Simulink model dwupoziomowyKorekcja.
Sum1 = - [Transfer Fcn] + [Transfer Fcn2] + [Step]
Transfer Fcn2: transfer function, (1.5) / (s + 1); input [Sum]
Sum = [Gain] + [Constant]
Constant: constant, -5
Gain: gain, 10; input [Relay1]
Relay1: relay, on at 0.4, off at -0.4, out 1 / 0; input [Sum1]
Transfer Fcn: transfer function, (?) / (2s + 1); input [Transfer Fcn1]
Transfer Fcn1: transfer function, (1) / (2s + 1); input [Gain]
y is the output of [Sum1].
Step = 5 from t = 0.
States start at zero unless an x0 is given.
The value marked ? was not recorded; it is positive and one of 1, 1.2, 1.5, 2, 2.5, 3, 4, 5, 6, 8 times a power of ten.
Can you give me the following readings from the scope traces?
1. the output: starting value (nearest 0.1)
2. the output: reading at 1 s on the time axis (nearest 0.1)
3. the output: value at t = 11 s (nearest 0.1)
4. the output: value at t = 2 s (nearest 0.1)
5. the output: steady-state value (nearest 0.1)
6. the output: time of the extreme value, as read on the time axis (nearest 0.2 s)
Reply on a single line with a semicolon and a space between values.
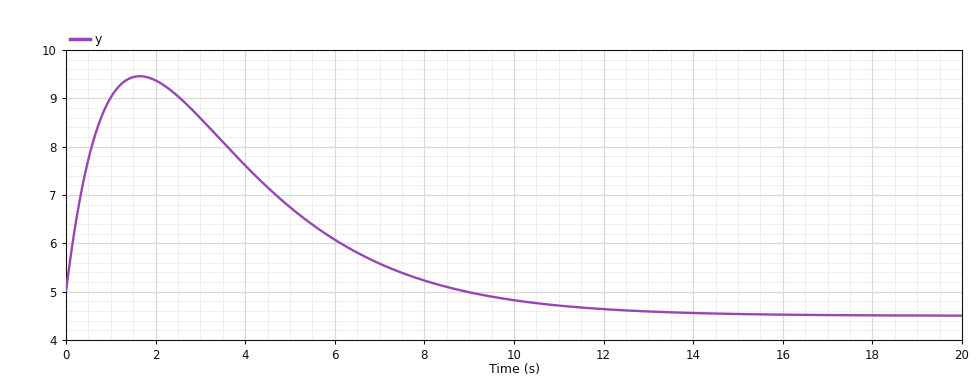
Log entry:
5.0; 9.0; 4.7; 9.4; 4.5; 1.6 s
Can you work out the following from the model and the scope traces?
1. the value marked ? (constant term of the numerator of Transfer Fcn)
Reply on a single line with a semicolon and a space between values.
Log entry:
0.8
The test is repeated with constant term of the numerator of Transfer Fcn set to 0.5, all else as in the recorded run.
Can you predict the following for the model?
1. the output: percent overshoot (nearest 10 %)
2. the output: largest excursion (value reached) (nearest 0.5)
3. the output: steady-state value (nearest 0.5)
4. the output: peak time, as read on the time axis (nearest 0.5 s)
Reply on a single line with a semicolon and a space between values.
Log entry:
110 %; 10.0; 7.5; 2.0 s
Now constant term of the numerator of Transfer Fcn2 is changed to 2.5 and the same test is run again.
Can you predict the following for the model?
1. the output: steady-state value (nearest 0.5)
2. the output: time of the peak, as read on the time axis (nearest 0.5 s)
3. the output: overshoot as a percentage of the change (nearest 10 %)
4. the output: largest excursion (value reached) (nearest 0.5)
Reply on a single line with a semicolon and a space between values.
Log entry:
9.5; 2.0 s; 90 %; 13.5
